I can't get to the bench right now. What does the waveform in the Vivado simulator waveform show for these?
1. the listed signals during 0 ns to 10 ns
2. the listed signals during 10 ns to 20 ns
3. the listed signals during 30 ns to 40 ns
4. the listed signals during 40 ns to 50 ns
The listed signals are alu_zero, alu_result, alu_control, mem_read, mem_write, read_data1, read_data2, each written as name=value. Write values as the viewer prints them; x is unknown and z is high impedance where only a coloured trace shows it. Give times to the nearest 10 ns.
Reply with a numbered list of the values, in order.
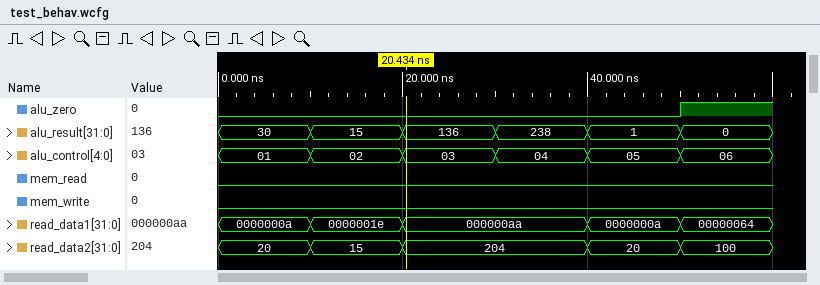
1. alu_zero=0, alu_result=30, alu_control=01, mem_read=0, mem_write=0, read_data1=0000000a, read_data2=20
2. alu_zero=0, alu_result=15, alu_control=02, mem_read=0, mem_write=0, read_data1=0000001e, read_data2=15
3. alu_zero=0, alu_result=238, alu_control=04, mem_read=0, mem_write=0, read_data1=000000aa, read_data2=204
4. alu_zero=0, alu_result=1, alu_control=05, mem_read=0, mem_write=0, read_data1=0000000a, read_data2=20
